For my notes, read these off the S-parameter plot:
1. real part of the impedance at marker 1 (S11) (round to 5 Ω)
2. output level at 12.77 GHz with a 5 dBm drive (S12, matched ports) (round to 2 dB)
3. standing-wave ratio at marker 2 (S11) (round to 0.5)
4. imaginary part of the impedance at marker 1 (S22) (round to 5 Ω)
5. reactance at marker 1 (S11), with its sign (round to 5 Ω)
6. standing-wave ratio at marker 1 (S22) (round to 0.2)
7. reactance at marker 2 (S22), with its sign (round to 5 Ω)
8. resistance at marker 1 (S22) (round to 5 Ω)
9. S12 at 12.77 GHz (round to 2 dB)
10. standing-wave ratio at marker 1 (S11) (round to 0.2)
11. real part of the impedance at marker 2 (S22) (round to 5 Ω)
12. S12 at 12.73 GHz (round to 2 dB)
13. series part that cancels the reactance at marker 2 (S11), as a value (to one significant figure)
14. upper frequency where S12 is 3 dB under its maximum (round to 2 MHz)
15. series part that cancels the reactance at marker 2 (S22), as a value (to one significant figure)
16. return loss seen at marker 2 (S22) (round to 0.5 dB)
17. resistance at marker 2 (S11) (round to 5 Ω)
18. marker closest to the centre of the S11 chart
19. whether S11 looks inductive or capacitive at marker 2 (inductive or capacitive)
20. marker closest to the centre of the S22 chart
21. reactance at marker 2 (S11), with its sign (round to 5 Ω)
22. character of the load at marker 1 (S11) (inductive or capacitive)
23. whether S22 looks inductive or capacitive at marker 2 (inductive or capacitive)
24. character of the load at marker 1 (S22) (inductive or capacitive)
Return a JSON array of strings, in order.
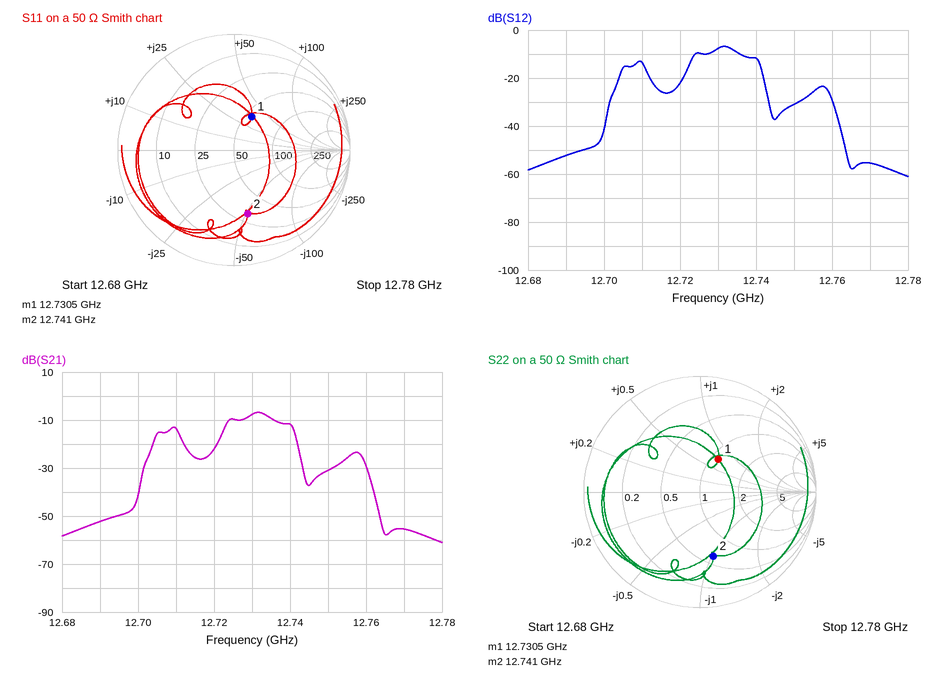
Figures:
["55 Ω", "-50 dBm", "3.5", "+35 Ω", "+35 Ω", "2.0", "-50 Ω", "55 Ω", "-56 dB", "2.0", "30 Ω", "-8 dB", "600 pH", "12.736 GHz", "600 pH", "5.0 dB", "30 Ω", "marker 1", "capacitive", "marker 1", "-50 Ω", "inductive", "capacitive", "inductive"]
